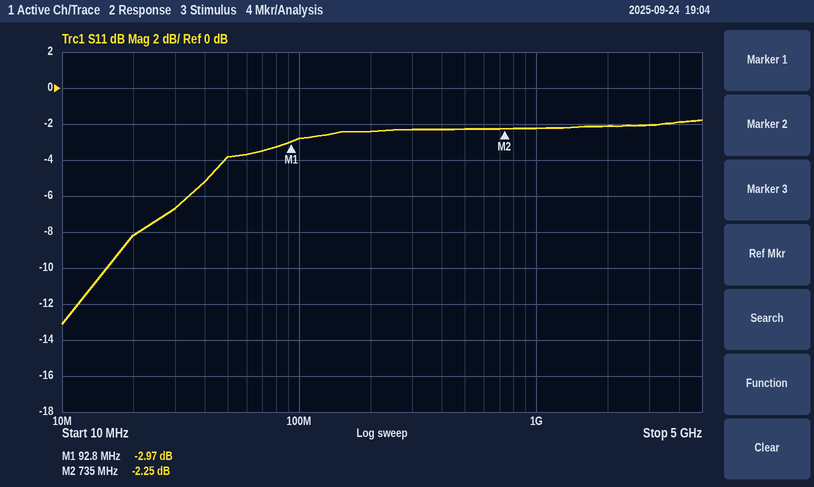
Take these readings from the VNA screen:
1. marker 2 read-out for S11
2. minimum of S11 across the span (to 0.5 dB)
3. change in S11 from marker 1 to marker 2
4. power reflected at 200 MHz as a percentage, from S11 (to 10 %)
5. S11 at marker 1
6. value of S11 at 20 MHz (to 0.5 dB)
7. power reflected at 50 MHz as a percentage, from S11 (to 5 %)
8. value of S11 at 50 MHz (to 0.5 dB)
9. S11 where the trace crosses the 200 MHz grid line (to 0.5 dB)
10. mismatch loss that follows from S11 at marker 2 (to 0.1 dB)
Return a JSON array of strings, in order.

["-2.25 dB", "-13.0 dB", "0.72 dB", "60 %", "-2.97 dB", "-8.0 dB", "40 %", "-4.0 dB", "-2.5 dB", "3.9 dB"]
